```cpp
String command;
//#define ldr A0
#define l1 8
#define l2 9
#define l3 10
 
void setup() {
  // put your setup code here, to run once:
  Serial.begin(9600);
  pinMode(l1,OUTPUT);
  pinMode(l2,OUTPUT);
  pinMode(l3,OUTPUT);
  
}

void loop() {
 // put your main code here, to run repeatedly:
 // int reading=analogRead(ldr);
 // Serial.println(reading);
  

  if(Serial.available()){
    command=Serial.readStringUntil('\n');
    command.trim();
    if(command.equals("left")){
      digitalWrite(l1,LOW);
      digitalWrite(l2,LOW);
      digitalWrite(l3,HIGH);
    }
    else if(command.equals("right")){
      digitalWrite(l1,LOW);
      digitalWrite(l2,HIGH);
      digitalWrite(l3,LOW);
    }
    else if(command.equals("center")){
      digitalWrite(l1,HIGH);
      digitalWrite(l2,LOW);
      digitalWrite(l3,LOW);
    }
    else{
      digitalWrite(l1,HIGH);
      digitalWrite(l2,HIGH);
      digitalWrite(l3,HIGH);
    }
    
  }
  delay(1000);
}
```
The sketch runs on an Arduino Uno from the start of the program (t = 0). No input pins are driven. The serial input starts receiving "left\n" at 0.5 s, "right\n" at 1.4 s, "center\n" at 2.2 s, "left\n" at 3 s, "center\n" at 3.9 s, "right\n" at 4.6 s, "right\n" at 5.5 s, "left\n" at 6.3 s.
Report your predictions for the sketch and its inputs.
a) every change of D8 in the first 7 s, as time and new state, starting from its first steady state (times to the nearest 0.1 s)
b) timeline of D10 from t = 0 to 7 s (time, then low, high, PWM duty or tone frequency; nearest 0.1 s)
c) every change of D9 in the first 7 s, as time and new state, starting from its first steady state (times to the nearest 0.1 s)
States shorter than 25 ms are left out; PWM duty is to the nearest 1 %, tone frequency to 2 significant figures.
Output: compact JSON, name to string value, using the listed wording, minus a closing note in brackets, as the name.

{"every change of D8 in the first 7 s, as time and new state, starting from its first steady state": "0 s low; 3 s high; 4 s low; 5 s high; 6 s low", "timeline of D10 from t = 0 to 7 s": "0 s low; 1 s high; 2 s low; 4 s high; 5 s low", "every change of D9 in the first 7 s, as time and new state, starting from its first steady state": "0 s low; 2 s high; 3 s low; 6 s high"}
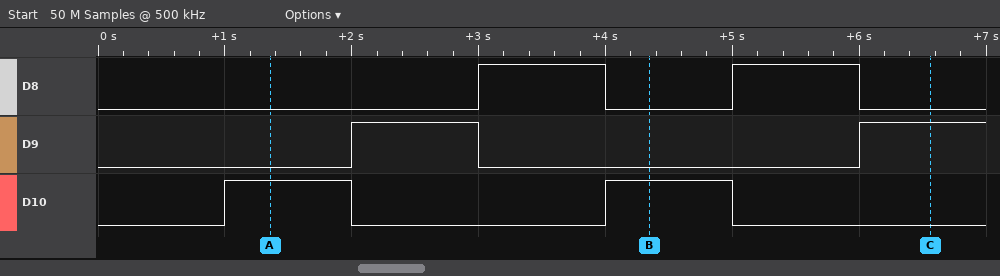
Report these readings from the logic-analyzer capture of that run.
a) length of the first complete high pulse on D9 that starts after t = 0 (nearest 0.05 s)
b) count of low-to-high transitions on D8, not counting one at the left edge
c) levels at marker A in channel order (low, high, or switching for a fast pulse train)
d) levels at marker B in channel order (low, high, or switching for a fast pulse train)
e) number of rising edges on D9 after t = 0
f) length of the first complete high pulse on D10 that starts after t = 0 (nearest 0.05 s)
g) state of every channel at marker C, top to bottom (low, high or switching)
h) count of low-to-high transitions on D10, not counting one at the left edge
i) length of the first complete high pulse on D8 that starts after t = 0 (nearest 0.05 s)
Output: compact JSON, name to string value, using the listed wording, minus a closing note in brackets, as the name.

{"length of the first complete high pulse on D9 that starts after t = 0": "1.00 s", "count of low-to-high transitions on D8, not counting one at the left edge": "2", "levels at marker A in channel order": "D8 low, D9 low, D10 high", "levels at marker B in channel order": "D8 low, D9 low, D10 high", "number of rising edges on D9 after t = 0": "2", "length of the first complete high pulse on D10 that starts after t = 0": "1.00 s", "state of every channel at marker C, top to bottom": "D8 low, D9 high, D10 low", "count of low-to-high transitions on D10, not counting one at the left edge": "2", "length of the first complete high pulse on D8 that starts after t = 0": "1.00 s"}
